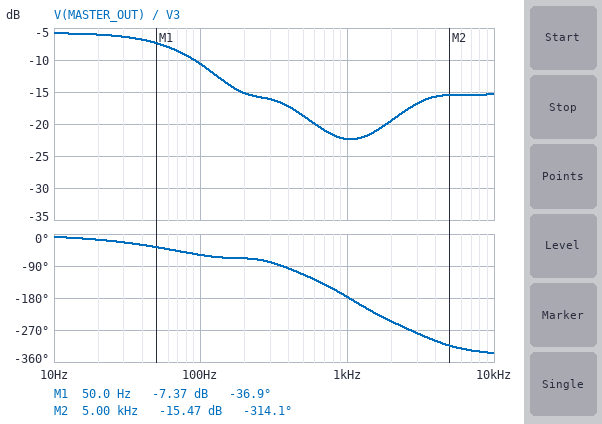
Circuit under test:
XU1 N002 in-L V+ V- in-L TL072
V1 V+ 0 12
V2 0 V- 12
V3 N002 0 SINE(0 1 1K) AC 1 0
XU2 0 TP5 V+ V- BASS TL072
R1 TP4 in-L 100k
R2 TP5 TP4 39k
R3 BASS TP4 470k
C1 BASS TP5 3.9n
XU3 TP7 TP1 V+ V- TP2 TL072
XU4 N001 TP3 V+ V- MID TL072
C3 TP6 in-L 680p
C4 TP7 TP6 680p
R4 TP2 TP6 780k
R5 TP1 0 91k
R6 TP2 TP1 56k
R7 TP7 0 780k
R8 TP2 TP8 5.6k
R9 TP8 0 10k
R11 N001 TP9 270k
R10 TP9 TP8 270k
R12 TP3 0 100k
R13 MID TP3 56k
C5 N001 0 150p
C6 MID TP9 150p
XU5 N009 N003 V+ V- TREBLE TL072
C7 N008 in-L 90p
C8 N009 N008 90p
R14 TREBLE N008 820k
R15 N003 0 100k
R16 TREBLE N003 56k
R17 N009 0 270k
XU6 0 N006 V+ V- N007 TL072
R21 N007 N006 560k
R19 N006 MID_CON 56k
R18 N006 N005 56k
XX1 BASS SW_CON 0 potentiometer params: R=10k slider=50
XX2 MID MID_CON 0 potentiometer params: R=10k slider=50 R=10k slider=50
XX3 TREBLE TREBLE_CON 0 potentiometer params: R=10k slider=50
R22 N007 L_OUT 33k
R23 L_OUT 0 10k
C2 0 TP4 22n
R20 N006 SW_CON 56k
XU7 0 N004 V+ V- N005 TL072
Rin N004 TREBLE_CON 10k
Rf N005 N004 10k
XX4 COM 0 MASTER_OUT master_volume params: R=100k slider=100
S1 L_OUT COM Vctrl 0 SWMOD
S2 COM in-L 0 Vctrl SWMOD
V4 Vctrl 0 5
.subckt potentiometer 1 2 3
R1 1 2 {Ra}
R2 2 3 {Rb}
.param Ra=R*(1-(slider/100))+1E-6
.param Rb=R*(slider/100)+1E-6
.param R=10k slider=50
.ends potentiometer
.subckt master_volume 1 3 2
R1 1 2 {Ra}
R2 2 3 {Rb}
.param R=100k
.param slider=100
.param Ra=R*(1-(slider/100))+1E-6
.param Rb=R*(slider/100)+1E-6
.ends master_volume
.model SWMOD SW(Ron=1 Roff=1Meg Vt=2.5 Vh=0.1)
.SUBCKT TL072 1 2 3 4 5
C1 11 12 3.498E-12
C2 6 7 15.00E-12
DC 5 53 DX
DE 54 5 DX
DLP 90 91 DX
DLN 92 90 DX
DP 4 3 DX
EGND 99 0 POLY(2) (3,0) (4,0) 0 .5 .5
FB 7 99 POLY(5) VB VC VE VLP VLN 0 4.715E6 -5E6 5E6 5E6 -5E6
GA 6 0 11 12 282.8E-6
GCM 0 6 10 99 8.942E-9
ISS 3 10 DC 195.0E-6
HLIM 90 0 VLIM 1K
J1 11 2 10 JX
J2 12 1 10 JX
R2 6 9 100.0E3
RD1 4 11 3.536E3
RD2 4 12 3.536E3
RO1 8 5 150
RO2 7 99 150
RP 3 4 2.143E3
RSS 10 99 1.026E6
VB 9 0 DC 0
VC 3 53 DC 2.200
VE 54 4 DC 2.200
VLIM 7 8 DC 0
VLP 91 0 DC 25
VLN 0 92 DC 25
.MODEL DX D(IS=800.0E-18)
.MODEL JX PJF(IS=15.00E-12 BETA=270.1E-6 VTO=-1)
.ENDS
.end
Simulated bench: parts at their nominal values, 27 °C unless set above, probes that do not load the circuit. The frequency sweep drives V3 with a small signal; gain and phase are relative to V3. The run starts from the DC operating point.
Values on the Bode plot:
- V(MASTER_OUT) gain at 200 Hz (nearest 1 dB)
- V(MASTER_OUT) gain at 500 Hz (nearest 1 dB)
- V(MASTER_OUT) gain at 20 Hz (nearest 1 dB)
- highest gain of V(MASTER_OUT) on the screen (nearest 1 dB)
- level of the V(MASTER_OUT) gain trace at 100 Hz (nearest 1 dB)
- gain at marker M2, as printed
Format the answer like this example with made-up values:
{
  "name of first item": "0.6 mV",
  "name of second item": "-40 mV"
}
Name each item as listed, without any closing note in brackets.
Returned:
{
  "V(MASTER_OUT) gain at 200 Hz": "-15 dB",
  "V(MASTER_OUT) gain at 500 Hz": "-19 dB",
  "V(MASTER_OUT) gain at 20 Hz": "-6 dB",
  "highest gain of V(MASTER_OUT) on the screen": "-6 dB",
  "level of the V(MASTER_OUT) gain trace at 100 Hz": "-11 dB",
  "gain at marker M2, as printed": "-15.47 dB"
}
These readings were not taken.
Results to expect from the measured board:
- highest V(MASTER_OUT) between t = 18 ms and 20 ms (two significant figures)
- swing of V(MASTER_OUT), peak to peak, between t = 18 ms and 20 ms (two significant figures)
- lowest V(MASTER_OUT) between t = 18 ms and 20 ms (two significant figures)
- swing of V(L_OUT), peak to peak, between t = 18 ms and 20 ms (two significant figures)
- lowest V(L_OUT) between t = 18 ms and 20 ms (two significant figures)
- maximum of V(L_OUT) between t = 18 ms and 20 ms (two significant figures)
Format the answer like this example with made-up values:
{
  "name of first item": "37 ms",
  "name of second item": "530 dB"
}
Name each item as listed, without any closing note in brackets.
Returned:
{
  "highest V(MASTER_OUT) between t = 18 ms and 20 ms": "1.8 V",
  "swing of V(MASTER_OUT), peak to peak, between t = 18 ms and 20 ms": "3.5 V",
  "lowest V(MASTER_OUT) between t = 18 ms and 20 ms": "-1.8 V",
  "swing of V(L_OUT), peak to peak, between t = 18 ms and 20 ms": "3.5 V",
  "lowest V(L_OUT) between t = 18 ms and 20 ms": "-1.8 V",
  "maximum of V(L_OUT) between t = 18 ms and 20 ms": "1.8 V"
}
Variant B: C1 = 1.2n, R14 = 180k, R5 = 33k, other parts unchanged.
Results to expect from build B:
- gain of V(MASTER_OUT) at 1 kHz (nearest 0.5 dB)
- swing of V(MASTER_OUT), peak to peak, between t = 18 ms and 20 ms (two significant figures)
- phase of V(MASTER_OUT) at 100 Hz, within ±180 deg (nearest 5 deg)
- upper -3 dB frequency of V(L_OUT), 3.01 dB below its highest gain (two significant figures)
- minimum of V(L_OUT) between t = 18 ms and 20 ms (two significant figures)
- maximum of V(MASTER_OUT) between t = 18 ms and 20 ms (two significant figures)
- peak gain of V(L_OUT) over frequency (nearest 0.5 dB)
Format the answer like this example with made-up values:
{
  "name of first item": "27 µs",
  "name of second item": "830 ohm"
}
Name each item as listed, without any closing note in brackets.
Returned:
{
  "gain of V(MASTER_OUT) at 1 kHz": "-13.5 dB",
  "swing of V(MASTER_OUT), peak to peak, between t = 18 ms and 20 ms": "4.5 V",
  "phase of V(MASTER_OUT) at 100 Hz, within ±180 deg": "-25 deg",
  "upper -3 dB frequency of V(L_OUT), 3.01 dB below its highest gain": "370 Hz",
  "minimum of V(L_OUT) between t = 18 ms and 20 ms": "-2.2 V",
  "maximum of V(MASTER_OUT) between t = 18 ms and 20 ms": "2.2 V",
  "peak gain of V(L_OUT) over frequency": "22.0 dB"
}
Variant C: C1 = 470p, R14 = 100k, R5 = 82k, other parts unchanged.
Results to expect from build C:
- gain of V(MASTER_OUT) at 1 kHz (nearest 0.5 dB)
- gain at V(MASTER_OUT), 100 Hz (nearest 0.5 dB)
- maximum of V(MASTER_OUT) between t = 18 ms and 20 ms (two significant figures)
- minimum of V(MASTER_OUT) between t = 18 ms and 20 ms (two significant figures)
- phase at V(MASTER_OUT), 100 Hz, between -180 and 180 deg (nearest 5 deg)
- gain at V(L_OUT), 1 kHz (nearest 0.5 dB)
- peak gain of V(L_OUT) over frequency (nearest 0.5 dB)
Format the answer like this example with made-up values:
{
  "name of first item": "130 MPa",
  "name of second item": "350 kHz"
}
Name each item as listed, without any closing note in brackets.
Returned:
{
  "gain of V(MASTER_OUT) at 1 kHz": "-17.5 dB",
  "gain at V(MASTER_OUT), 100 Hz": "-5.0 dB",
  "maximum of V(MASTER_OUT) between t = 18 ms and 20 ms": "2.2 V",
  "minimum of V(MASTER_OUT) between t = 18 ms and 20 ms": "-2.2 V",
  "phase at V(MASTER_OUT), 100 Hz, between -180 and 180 deg": "-10 deg",
  "gain at V(L_OUT), 1 kHz": "8.5 dB",
  "peak gain of V(L_OUT) over frequency": "19.0 dB"
}
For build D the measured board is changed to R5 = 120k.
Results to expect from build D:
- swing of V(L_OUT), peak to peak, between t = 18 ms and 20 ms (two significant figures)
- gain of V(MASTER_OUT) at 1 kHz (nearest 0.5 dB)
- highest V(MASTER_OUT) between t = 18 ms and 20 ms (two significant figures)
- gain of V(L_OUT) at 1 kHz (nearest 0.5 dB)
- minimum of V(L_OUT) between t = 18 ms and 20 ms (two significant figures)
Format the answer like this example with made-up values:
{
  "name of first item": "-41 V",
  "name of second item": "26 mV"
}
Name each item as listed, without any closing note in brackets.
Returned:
{
  "swing of V(L_OUT), peak to peak, between t = 18 ms and 20 ms": "3.2 V",
  "gain of V(MASTER_OUT) at 1 kHz": "-24.5 dB",
  "highest V(MASTER_OUT) between t = 18 ms and 20 ms": "1.6 V",
  "gain of V(L_OUT) at 1 kHz": "4.5 dB",
  "minimum of V(L_OUT) between t = 18 ms and 20 ms": "-1.6 V"
}
